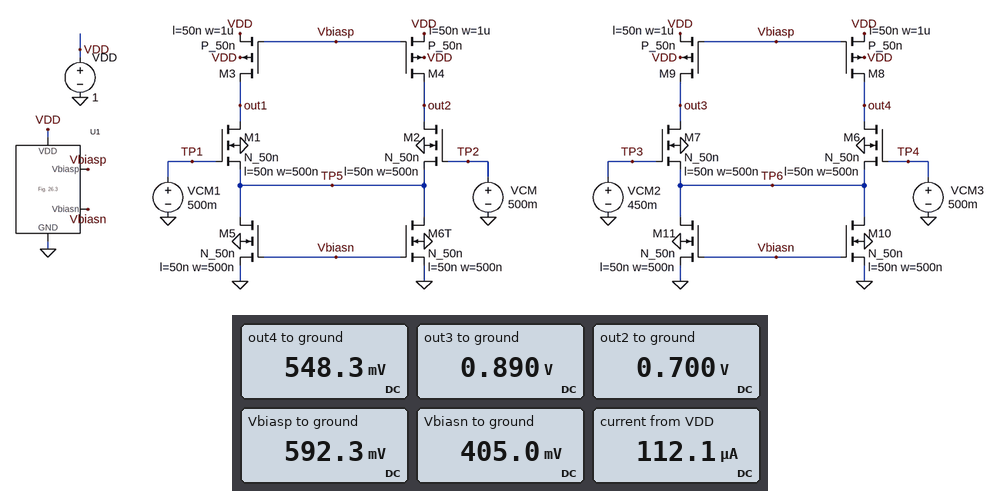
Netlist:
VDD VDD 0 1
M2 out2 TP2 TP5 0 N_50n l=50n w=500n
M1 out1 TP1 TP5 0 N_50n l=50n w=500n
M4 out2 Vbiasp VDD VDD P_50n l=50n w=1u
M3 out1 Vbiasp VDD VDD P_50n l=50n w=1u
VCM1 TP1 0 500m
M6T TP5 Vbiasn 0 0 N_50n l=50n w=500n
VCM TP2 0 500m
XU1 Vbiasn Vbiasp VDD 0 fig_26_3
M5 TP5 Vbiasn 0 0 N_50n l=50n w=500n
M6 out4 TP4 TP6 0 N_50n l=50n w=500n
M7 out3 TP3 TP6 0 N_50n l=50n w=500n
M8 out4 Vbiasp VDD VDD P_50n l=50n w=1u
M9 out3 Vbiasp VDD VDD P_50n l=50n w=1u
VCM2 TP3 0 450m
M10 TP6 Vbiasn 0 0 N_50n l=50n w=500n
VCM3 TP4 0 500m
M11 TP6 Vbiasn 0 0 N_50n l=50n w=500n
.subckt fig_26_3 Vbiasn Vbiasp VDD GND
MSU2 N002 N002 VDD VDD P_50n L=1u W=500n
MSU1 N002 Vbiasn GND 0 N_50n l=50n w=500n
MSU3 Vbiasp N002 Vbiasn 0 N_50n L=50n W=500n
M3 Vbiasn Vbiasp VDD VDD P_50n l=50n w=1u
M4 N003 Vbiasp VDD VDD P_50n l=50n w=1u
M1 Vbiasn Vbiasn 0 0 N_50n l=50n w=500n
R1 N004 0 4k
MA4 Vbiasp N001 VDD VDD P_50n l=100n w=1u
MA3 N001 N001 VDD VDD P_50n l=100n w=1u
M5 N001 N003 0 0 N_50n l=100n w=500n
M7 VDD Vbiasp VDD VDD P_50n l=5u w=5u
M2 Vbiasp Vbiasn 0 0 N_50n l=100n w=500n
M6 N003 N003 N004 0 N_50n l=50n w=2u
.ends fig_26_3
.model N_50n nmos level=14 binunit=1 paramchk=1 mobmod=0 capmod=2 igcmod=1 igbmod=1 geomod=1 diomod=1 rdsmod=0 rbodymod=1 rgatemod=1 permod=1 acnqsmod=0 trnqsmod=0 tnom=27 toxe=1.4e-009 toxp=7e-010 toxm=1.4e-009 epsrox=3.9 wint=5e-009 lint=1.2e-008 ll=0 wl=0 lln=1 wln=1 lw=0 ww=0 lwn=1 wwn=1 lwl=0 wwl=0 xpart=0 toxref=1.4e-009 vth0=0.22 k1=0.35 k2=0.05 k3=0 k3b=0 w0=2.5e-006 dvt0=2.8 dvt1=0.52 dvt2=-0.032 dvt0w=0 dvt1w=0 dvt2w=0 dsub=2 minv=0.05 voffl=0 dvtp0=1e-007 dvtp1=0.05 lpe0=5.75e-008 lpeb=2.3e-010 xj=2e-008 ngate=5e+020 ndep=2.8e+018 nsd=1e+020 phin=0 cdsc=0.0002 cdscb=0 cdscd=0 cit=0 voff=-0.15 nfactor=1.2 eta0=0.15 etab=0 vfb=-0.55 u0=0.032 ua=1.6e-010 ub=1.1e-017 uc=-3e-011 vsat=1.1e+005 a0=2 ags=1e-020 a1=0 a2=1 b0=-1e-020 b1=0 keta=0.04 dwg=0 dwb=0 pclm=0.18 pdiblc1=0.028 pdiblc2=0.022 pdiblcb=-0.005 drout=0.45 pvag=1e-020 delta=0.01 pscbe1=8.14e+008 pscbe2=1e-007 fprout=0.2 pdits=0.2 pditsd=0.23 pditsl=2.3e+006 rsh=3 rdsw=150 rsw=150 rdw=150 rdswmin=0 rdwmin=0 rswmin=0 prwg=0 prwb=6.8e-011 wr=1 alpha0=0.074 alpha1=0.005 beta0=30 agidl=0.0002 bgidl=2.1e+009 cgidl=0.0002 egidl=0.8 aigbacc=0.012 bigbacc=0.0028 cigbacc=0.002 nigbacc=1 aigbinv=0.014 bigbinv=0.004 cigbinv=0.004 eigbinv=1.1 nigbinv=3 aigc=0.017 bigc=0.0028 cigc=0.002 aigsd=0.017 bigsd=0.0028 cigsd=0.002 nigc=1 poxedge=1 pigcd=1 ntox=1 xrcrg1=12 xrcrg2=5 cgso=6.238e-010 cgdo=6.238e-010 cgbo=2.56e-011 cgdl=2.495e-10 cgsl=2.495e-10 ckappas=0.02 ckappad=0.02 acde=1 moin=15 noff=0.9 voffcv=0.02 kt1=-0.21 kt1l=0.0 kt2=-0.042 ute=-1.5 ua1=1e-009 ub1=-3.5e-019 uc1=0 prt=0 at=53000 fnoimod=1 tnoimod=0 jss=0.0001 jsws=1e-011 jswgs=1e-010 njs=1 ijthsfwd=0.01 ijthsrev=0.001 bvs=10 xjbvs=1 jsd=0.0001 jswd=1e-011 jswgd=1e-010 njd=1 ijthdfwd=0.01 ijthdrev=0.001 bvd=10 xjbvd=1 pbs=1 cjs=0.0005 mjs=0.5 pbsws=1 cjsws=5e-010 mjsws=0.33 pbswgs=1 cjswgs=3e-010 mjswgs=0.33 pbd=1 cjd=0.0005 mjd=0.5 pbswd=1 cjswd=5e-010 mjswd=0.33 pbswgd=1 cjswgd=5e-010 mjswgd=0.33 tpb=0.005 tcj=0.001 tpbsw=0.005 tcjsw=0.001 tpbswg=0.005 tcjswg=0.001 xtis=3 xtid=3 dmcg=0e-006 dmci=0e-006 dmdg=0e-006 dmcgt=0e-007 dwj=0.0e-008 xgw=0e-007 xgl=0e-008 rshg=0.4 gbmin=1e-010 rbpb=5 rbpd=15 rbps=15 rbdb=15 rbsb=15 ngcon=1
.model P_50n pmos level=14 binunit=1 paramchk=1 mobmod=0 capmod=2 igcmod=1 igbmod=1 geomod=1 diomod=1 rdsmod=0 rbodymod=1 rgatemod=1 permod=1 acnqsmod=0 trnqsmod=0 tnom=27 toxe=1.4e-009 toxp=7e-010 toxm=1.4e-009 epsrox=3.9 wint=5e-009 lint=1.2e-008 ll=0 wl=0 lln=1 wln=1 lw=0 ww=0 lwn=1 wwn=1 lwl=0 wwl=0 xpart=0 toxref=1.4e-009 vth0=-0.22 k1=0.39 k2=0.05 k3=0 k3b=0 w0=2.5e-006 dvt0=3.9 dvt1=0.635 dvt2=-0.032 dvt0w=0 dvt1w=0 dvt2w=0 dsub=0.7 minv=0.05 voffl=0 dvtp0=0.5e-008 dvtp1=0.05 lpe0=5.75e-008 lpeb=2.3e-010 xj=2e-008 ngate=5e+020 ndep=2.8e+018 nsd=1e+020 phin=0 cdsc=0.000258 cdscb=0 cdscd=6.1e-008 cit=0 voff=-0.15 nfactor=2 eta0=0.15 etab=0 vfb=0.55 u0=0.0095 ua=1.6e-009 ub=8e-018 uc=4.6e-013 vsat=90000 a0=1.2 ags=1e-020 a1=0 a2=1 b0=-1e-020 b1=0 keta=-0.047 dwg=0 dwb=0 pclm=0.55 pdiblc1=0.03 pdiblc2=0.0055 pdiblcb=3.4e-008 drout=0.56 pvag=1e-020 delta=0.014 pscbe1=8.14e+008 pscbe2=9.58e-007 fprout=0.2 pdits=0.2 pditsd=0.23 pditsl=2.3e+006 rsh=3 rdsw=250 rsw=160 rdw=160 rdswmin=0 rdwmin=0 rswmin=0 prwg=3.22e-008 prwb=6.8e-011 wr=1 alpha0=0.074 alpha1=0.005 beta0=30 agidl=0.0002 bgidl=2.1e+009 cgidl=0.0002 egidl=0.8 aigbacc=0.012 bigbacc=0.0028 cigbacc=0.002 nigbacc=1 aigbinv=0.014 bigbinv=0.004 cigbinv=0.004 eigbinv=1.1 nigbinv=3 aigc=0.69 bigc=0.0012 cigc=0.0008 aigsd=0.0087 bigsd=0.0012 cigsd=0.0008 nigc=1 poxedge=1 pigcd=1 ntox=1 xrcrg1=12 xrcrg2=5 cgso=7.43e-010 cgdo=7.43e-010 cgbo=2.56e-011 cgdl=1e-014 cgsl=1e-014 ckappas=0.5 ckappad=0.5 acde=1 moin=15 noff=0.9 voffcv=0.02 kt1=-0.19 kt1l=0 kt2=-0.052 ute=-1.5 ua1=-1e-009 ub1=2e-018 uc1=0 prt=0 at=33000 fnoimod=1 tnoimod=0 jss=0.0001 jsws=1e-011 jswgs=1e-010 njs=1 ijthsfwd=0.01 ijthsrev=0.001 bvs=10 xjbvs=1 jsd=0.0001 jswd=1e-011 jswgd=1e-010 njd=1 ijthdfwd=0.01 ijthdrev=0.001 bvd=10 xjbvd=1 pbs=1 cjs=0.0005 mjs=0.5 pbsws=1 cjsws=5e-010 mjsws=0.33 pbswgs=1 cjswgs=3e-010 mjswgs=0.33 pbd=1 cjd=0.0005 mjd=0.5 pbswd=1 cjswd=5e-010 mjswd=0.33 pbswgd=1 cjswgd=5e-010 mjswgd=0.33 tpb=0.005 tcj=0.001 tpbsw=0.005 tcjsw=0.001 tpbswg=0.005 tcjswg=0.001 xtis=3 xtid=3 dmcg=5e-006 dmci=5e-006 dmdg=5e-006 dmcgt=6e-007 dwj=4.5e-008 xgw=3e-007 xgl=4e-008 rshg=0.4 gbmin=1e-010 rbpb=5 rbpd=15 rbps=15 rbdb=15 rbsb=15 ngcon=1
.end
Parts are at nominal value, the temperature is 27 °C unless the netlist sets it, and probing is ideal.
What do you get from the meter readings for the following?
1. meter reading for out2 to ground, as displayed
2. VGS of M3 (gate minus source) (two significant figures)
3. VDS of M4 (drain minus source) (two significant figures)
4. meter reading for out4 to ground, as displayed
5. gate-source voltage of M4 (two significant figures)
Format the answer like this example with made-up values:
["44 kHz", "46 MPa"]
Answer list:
["0.700 V", "-410 mV", "-300 mV", "548.3 mV", "-410 mV"]
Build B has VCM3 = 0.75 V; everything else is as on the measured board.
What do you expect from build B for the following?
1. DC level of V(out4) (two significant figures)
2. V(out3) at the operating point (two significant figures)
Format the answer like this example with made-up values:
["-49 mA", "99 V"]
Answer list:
["170 mV", "960 mV"]
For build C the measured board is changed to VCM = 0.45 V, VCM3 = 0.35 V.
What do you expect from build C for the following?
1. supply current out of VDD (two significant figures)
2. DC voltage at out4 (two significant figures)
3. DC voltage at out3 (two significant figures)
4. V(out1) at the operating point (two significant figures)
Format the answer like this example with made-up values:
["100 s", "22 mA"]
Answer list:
["100 µA", "970 mV", "570 mV", "550 mV"]
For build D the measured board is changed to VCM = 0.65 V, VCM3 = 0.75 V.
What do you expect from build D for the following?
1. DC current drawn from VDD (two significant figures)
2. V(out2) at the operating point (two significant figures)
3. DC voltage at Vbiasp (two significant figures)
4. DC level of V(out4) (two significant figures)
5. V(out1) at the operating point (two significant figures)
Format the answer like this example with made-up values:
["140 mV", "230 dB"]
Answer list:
["120 µA", "230 mV", "590 mV", "170 mV", "930 mV"]
